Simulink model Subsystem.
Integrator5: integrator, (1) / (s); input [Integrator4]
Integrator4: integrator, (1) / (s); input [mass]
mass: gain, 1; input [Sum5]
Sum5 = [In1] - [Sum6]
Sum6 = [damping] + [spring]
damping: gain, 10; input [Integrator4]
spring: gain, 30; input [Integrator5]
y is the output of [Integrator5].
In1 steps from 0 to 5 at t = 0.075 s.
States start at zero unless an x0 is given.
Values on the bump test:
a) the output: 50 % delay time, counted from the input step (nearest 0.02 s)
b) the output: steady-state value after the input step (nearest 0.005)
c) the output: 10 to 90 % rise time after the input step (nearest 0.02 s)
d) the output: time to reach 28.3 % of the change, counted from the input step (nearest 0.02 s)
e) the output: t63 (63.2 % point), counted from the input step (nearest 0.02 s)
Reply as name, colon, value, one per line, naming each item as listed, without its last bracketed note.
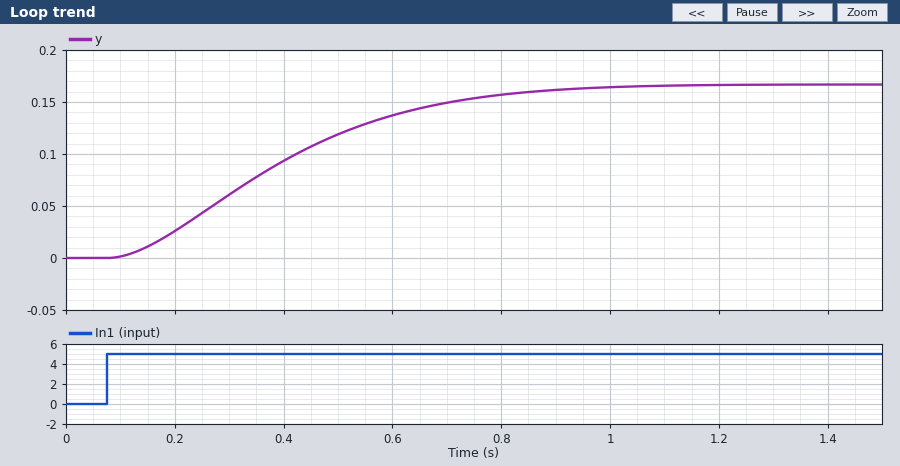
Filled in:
the output: 50 % delay time, counted from the input step: 0.30 s
the output: steady-state value after the input step: 0.165
the output: 10 to 90 % rise time after the input step: 0.54 s
the output: time to reach 28.3 % of the change, counted from the input step: 0.18 s
the output: t63 (63.2 % point), counted from the input step: 0.36 s
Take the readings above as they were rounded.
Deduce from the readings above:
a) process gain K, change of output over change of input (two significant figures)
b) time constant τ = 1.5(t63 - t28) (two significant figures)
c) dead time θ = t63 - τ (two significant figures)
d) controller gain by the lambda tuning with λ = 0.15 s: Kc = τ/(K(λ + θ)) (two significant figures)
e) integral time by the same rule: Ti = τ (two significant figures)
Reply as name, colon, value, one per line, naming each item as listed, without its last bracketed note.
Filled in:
process gain K, change of output over change of input: 0.033
time constant τ = 1.5(t63 - t28): 0.27 s
dead time θ = t63 - τ: 0.090 s
controller gain by the lambda tuning with λ = 0.15 s: Kc = τ/(K(λ + θ)): 34
integral time by the same rule: Ti = τ: 0.27 s
